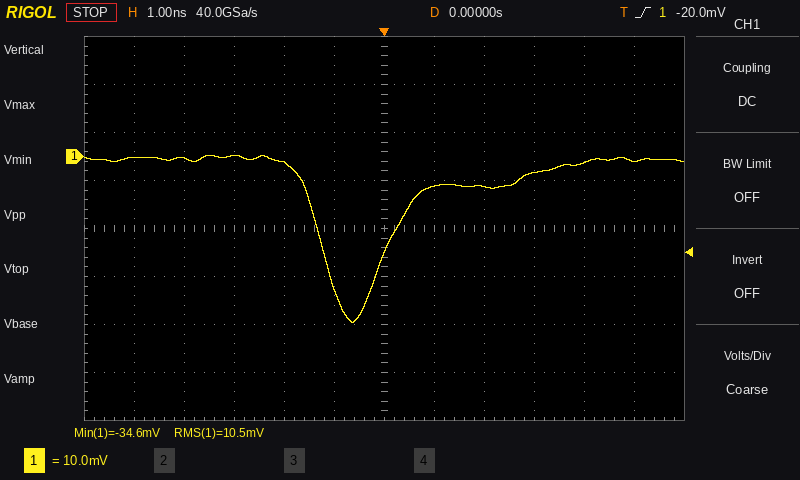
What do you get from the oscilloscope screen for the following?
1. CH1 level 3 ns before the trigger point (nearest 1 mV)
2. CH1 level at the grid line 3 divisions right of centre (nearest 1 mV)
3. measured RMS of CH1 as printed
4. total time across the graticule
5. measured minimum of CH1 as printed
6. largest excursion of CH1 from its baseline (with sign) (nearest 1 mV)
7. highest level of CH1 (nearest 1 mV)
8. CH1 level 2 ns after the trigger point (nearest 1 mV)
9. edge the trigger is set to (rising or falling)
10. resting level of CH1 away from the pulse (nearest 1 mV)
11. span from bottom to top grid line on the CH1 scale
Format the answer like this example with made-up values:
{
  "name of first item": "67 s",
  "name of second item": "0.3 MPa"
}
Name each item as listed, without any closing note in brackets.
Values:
{
  "CH1 level 3 ns before the trigger point": "0 mV",
  "CH1 level at the grid line 3 divisions right of centre": "-3 mV",
  "measured RMS of CH1 as printed": "10.5 mV",
  "total time across the graticule": "12 ns",
  "measured minimum of CH1 as printed": "-34.6 mV",
  "largest excursion of CH1 from its baseline (with sign)": "-34 mV",
  "highest level of CH1": "0 mV",
  "CH1 level 2 ns after the trigger point": "-6 mV",
  "edge the trigger is set to": "rising",
  "resting level of CH1 away from the pulse": "-1 mV",
  "span from bottom to top grid line on the CH1 scale": "80 mV"
}
